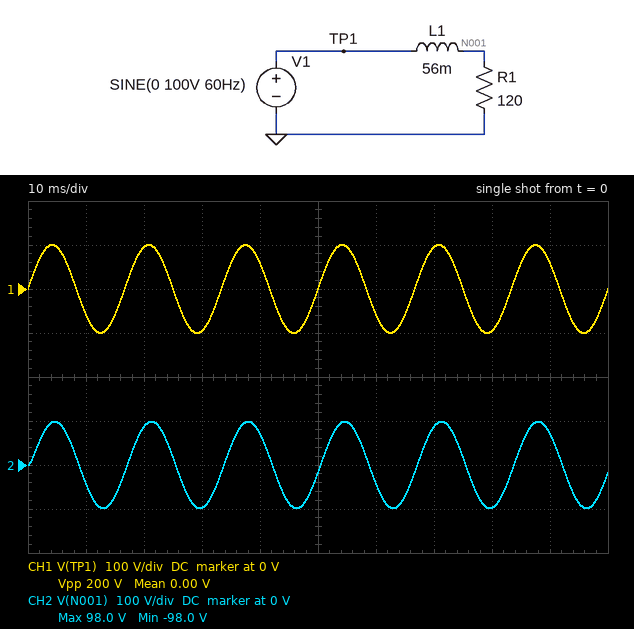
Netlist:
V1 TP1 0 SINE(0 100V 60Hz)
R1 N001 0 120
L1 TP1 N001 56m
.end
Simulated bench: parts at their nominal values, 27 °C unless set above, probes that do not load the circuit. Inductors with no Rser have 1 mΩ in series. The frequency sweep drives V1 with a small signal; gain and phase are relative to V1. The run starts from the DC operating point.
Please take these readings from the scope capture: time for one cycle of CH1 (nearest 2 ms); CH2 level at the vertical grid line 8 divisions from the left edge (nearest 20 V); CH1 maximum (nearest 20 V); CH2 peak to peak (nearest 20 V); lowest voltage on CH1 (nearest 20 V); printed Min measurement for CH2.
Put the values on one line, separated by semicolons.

16 ms; -100 V; 100 V; 200 V; -100 V; -98.0 V
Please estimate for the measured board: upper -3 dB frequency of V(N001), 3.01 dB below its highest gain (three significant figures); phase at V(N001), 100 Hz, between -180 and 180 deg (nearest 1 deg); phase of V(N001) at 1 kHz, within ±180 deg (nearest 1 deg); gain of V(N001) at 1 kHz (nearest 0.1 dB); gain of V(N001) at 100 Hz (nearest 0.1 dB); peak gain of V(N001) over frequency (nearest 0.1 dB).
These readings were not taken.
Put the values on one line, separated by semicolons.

341 Hz; -16 deg; -71 deg; -9.8 dB; -0.4 dB; 0 dB
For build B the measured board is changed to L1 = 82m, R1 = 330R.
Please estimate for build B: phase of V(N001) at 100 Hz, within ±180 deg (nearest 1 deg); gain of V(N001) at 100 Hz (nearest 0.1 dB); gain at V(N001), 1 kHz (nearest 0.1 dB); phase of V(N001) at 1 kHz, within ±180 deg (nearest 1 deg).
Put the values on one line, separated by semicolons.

-9 deg; -0.1 dB; -5.4 dB; -57 deg
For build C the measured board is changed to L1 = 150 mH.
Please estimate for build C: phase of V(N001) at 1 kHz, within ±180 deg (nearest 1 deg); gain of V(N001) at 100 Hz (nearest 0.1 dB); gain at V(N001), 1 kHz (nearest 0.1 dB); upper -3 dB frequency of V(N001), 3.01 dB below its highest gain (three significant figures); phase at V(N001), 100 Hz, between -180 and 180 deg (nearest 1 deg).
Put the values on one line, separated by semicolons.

-83 deg; -2.1 dB; -18.0 dB; 127 Hz; -38 deg
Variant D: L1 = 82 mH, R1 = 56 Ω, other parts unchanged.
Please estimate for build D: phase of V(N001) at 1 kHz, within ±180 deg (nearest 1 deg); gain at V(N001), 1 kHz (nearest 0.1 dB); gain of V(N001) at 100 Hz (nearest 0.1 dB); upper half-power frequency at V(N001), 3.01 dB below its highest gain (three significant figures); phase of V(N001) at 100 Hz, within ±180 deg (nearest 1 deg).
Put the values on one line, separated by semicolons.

-84 deg; -19.3 dB; -2.7 dB; 109 Hz; -43 deg
